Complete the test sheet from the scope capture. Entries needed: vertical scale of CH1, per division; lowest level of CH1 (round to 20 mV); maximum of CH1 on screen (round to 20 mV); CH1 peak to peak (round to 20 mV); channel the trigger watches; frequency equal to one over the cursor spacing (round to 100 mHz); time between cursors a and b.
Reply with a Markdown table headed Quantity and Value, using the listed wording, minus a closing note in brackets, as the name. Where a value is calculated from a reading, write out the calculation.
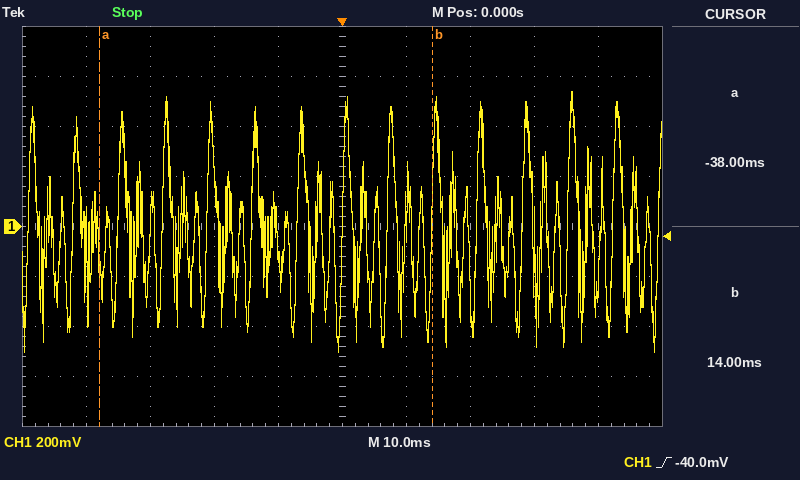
| Quantity | Value |
|---|---|
| vertical scale of CH1, per division | 200 mV |
| lowest level of CH1 | -500 mV |
| maximum of CH1 on screen | 540 mV |
| CH1 peak to peak | 540 mV − (-500 mV) = 1.04 V |
| channel the trigger watches | CH1 |
| frequency equal to one over the cursor spacing | 1 / 52 ms ≈ 19.2 Hz |
| time between cursors a and b | 14 ms − (-38 ms) = 52 ms |
